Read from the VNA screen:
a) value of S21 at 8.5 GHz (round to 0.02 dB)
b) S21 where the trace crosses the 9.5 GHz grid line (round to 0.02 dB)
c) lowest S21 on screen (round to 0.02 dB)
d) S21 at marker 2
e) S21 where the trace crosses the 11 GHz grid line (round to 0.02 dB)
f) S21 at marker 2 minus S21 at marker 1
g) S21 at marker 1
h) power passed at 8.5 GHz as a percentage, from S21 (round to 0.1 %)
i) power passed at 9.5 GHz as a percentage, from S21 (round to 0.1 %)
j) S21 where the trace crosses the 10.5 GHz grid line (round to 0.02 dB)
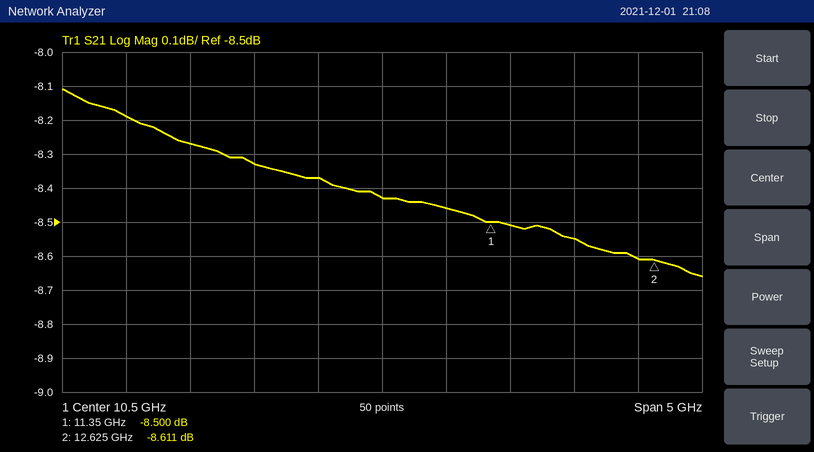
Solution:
-8.18 dB
-8.32 dB
-8.66 dB
-8.611 dB
-8.46 dB
-0.111 dB
-8.500 dB
15.2 %
14.7 %
-8.42 dB
